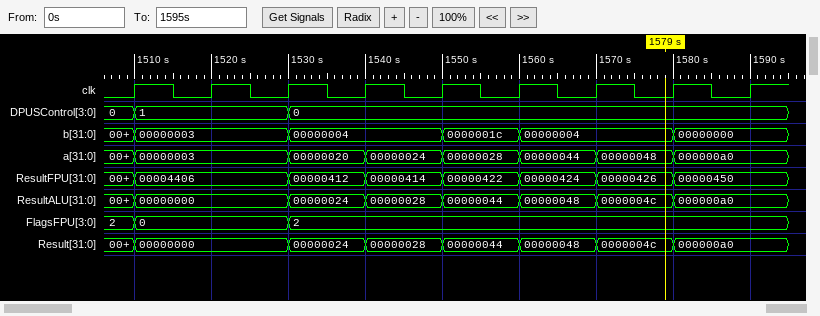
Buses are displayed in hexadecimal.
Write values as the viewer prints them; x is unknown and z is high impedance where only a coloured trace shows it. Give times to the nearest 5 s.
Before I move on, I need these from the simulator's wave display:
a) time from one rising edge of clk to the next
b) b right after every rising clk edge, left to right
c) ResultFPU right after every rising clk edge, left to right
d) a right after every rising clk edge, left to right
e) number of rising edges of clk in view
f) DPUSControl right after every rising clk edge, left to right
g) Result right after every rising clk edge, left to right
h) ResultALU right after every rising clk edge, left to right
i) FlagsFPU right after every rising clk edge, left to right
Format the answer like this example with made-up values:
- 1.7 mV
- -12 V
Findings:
- 10 s
- 00000003, 00000003, 00000004, 00000004, 0000001c, 00000004, 00000004, 00000000, 00000000
- 00004406, 00004406, 00000412, 00000414, 00000422, 00000424, 00000426, 00000450, 00000450
- 00000003, 00000003, 00000020, 00000024, 00000028, 00000044, 00000048, 000000a0, 000000a0
- 9
- 1, 1, 0, 0, 0, 0, 0, 0, 0
- 00000000, 00000000, 00000024, 00000028, 00000044, 00000048, 0000004c, 000000a0, 000000a0
- 00000000, 00000000, 00000024, 00000028, 00000044, 00000048, 0000004c, 000000a0, 000000a0
- 0, 0, 2, 2, 2, 2, 2, 2, 2
